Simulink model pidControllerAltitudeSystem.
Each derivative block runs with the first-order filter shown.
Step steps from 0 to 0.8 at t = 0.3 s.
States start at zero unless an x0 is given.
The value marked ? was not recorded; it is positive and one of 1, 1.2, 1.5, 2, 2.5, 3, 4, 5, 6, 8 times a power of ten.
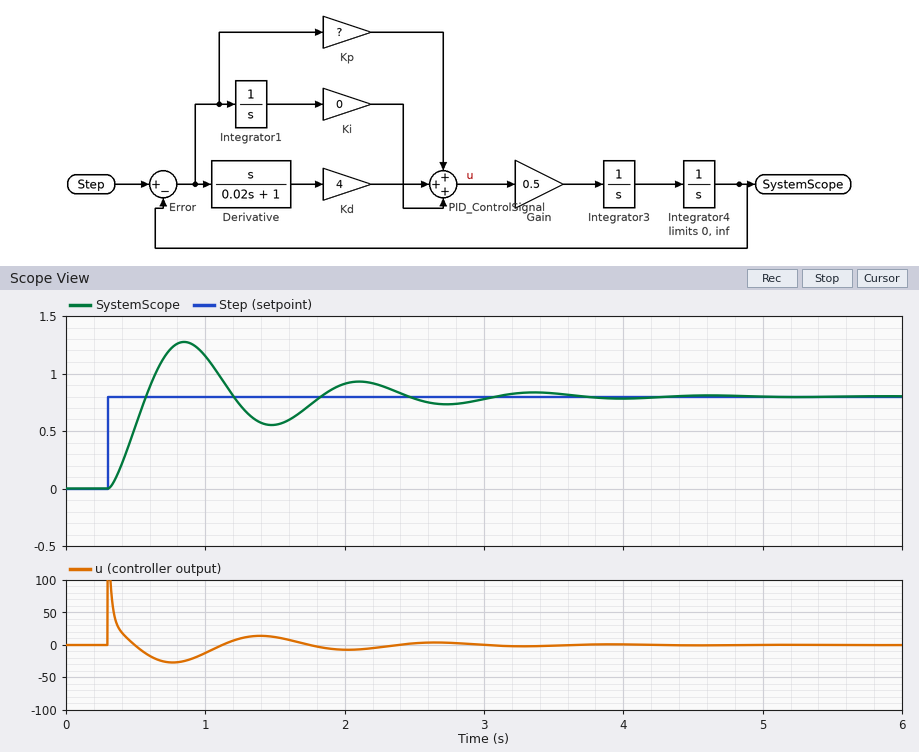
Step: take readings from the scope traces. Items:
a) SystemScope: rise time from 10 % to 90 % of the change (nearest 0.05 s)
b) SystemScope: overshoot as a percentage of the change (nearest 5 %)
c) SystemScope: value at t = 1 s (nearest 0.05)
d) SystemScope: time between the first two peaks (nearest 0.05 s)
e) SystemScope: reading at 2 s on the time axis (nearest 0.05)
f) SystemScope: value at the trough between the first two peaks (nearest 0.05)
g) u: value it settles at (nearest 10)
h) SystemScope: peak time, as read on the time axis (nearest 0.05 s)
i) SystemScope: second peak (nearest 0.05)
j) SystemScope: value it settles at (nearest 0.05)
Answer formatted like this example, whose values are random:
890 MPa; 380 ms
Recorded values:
0.20 s; 60 %; 1.15; 1.25 s; 0.90; 0.55; 0; 0.85 s; 0.95; 0.80
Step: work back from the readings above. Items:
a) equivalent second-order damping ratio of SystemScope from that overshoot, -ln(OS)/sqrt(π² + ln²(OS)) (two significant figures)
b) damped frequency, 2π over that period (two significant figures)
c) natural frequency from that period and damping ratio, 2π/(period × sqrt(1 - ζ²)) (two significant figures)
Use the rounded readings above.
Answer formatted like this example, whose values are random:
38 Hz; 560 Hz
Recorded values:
0.16; 5.0 rad/s; 5.1 rad/s
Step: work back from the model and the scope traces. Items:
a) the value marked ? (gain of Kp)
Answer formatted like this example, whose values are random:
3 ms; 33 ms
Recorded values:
50
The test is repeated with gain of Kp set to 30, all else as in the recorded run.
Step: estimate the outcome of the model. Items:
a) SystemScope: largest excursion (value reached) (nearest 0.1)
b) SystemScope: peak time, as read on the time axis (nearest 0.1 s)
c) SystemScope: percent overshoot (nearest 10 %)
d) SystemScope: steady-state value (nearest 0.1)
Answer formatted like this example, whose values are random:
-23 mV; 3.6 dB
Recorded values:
1.2; 1.0 s; 50 %; 0.8
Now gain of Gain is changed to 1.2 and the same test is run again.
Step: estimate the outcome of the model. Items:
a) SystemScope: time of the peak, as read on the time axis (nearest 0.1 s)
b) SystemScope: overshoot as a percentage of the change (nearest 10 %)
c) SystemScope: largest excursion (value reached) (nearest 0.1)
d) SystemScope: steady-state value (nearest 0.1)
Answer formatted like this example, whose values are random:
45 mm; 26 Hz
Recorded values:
0.6 s; 50 %; 1.2; 0.8
